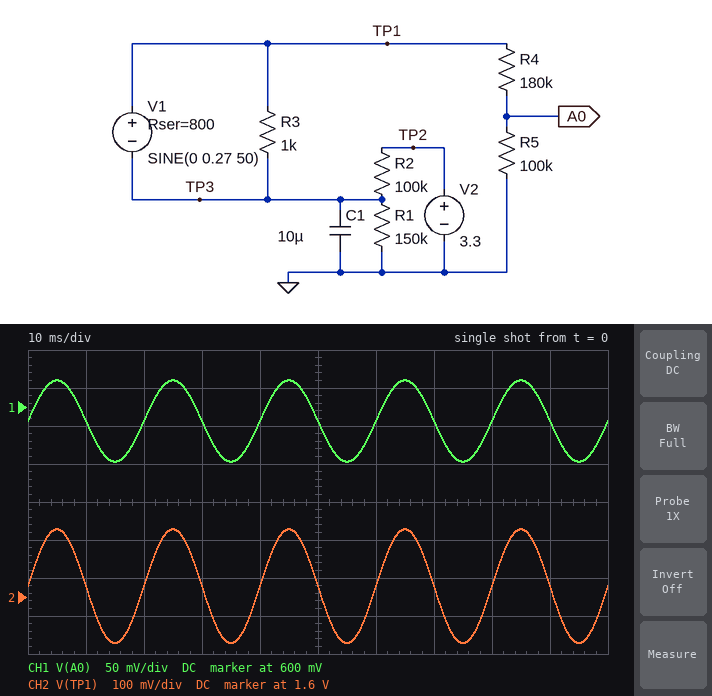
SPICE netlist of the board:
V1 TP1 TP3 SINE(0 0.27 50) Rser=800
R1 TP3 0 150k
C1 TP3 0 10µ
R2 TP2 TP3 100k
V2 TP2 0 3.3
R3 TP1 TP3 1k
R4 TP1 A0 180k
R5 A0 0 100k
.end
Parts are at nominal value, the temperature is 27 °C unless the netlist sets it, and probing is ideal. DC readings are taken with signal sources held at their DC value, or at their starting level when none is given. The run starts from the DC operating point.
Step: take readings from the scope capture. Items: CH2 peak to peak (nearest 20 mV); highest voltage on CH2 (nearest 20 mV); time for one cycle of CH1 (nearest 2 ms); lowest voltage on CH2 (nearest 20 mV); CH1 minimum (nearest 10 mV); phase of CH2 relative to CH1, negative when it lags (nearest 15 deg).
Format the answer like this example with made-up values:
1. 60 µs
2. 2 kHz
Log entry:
1. 300 mV
2. 1.78 V
3. 20 ms
4. 1.48 V
5. 530 mV
6. 0 deg
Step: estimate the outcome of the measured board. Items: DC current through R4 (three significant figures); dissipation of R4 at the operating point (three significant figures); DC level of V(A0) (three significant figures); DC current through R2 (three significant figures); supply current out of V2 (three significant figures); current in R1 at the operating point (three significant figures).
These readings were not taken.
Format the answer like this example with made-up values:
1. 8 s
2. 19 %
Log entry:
1. 5.82 µA
2. 6.09 µW
3. 582 mV
4. 16.7 µA
5. 16.7 µA
6. 10.9 µA
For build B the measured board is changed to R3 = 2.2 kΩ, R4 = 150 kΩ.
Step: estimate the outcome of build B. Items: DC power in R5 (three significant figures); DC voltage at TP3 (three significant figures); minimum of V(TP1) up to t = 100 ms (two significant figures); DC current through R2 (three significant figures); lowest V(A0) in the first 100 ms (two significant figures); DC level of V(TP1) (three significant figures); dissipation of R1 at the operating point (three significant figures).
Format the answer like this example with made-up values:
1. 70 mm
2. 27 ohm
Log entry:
1. 4.06 µW
2. 1.60 V
3. 1.4 V
4. 17.0 µA
5. 560 mV
6. 1.59 V
7. 17.0 µW
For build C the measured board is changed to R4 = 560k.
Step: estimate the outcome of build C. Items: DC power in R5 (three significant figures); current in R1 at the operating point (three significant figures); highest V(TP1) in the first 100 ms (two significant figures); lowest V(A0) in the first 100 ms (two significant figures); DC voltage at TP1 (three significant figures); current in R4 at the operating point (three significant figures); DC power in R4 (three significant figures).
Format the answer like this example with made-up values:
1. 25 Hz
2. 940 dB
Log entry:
1. 755 nW
2. 12.1 µA
3. 2.0 V
4. 250 mV
5. 1.81 V
6. 2.75 µA
7. 4.23 µW
